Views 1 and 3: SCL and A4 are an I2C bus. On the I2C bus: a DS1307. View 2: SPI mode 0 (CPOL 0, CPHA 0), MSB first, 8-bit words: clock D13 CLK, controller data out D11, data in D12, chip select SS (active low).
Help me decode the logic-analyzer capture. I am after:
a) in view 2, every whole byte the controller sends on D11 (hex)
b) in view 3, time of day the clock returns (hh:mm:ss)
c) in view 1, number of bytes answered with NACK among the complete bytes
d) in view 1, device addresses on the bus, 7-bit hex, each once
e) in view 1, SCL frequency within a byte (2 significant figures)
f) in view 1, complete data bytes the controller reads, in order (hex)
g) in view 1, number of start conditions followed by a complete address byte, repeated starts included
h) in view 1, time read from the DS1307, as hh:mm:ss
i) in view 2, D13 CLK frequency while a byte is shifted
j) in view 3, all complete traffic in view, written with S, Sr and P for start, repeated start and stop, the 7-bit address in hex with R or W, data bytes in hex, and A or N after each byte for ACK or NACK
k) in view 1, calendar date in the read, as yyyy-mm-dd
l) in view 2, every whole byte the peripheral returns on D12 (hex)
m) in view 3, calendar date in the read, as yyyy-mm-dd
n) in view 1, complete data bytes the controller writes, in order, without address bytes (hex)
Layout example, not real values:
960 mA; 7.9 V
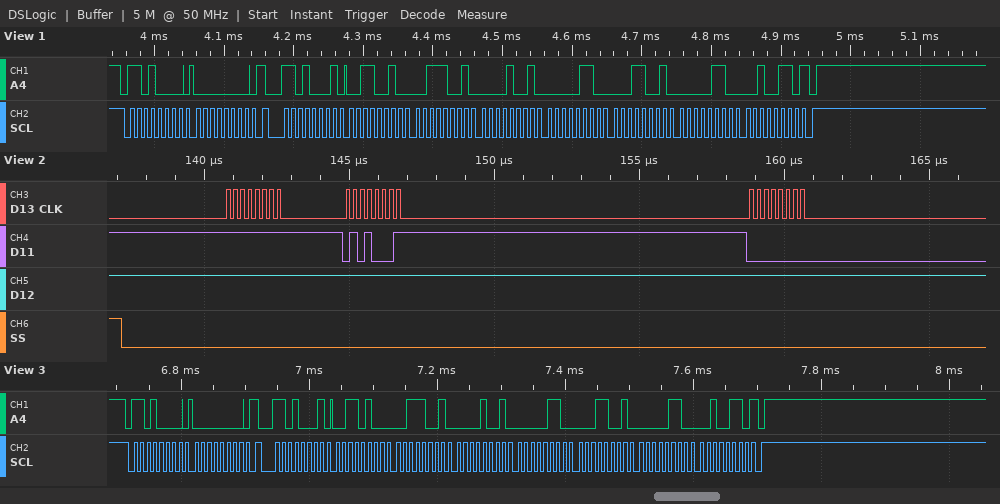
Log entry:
0xFF 0x51 0x00; 09:39:34; 1; 0x68; 100 kHz; 32 39 09 06 19 06 26; 2; 09:39:32; 4 MHz; S 68W A 00 A Sr 68R A 34 A 39 A 09 A 06 A 19 A 06 A 26 N P; 2026-06-19; 0xFF 0xFF 0xFF; 2026-06-19; 00
